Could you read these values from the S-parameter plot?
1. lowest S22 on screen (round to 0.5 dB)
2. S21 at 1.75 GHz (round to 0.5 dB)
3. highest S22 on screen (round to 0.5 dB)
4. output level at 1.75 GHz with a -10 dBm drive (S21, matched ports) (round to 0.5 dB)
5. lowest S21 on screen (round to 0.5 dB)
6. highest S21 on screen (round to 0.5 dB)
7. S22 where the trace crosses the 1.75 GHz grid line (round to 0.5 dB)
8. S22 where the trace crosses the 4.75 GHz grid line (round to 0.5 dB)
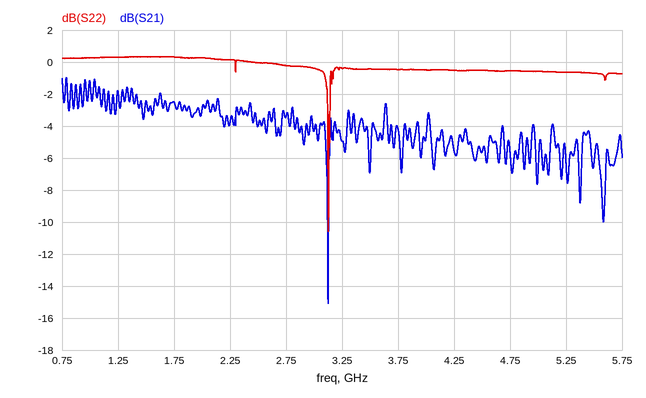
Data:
-10.5 dB
-2.5 dB
0.5 dB
-12.5 dBm
-15.0 dB
-1.0 dB
0.5 dB
-0.5 dB
